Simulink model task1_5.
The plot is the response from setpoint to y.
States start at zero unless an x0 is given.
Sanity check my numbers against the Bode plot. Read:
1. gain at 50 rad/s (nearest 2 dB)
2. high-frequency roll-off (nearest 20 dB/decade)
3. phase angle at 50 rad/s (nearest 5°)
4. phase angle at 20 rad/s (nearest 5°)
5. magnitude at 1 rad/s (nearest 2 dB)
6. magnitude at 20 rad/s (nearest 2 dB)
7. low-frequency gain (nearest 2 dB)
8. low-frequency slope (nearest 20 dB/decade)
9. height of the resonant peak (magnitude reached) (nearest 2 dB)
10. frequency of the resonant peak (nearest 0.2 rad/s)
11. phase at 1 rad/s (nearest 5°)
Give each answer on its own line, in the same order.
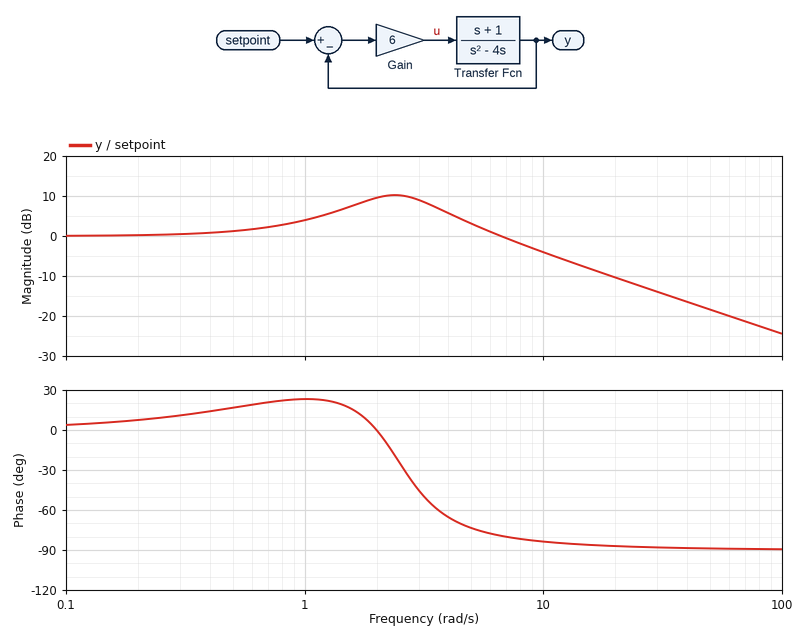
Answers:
-18 dB
-20 dB/decade
-90°
-85°
4 dB
-10 dB
0 dB
0 dB/decade
10 dB
2.4 rad/s
25°
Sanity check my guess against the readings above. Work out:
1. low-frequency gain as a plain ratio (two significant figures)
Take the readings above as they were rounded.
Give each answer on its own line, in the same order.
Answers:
1.0
